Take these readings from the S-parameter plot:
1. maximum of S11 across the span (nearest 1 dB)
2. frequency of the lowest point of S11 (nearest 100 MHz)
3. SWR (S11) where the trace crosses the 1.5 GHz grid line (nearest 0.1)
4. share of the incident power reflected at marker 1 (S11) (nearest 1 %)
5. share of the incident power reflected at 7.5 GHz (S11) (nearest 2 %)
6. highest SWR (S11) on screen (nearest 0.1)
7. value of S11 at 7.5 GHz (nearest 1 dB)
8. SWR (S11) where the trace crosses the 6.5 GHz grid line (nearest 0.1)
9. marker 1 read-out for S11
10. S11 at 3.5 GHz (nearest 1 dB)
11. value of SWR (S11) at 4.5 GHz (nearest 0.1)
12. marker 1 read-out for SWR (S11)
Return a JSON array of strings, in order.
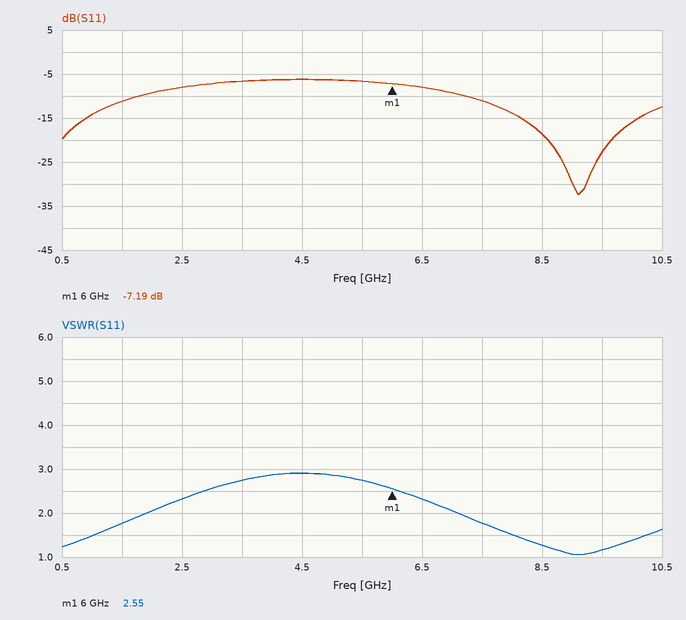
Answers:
["-6 dB", "9.1 GHz", "1.8", "19 %", "8 %", "2.9", "-11 dB", "2.3", "-7.19 dB", "-7 dB", "2.9", "2.55"]
